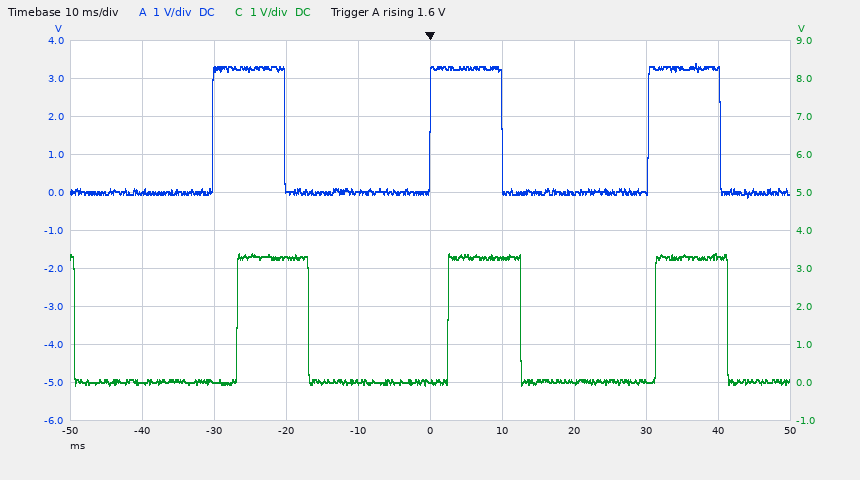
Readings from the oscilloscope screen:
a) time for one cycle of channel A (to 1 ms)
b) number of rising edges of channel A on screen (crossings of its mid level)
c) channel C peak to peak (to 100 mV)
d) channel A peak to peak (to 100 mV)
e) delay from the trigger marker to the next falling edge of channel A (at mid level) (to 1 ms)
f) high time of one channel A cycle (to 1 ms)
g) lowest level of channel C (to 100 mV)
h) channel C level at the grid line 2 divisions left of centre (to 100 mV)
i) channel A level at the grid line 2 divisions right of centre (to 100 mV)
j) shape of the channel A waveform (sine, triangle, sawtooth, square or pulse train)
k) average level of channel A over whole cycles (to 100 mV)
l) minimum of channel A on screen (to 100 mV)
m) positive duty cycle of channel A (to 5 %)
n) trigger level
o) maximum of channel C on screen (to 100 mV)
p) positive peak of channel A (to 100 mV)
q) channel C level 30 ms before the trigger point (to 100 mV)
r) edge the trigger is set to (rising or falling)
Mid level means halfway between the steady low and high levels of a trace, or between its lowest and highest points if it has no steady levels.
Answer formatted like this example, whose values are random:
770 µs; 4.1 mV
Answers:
30 ms; 3; 3.5 V; 3.5 V; 10 ms; 10 ms; -100 mV; 3.3 V; 0.0 V; pulse train; 1.1 V; -100 mV; 35 %; 1.6 V; 3.4 V; 3.4 V; 0.0 V; rising
